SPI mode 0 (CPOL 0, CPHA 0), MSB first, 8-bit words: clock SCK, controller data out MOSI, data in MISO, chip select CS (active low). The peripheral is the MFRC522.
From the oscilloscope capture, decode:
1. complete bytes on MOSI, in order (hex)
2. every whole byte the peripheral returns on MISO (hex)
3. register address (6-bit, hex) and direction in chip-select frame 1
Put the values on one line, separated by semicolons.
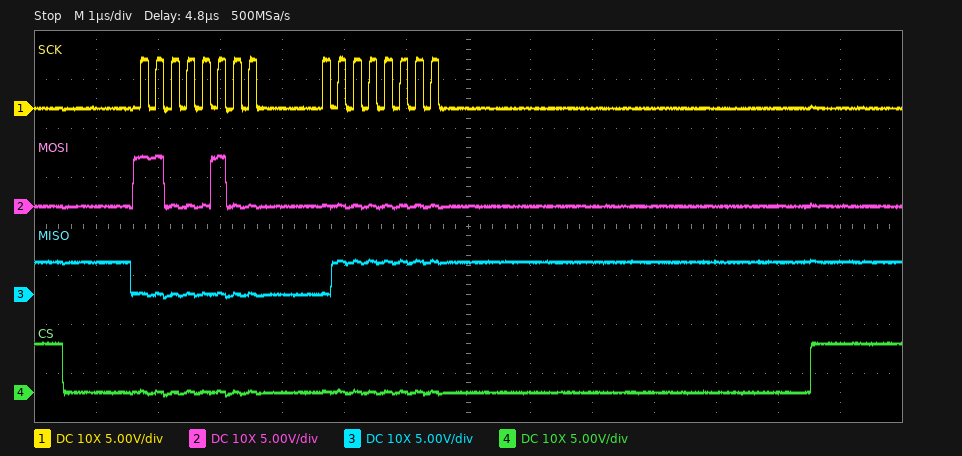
0xC4 0x00; 0x00 0x7F; 0x22 read
